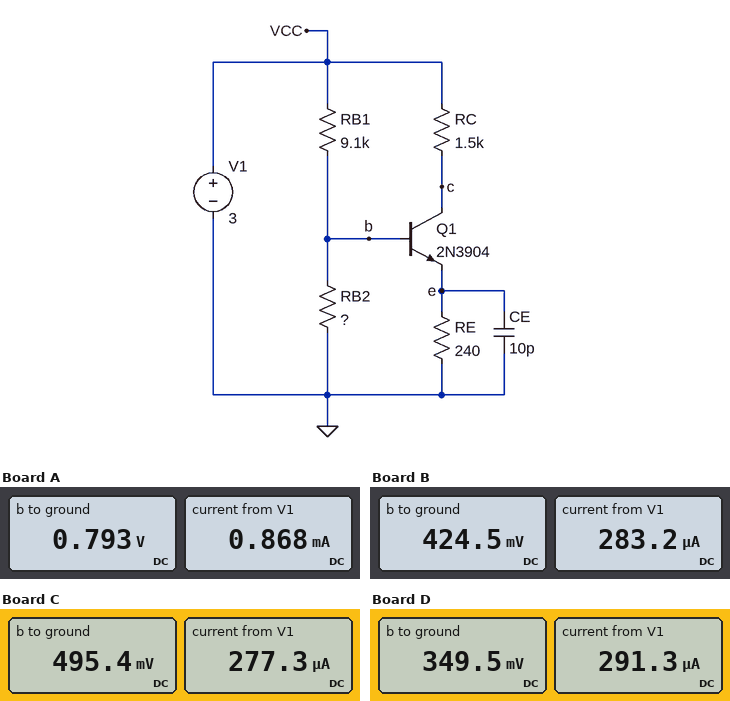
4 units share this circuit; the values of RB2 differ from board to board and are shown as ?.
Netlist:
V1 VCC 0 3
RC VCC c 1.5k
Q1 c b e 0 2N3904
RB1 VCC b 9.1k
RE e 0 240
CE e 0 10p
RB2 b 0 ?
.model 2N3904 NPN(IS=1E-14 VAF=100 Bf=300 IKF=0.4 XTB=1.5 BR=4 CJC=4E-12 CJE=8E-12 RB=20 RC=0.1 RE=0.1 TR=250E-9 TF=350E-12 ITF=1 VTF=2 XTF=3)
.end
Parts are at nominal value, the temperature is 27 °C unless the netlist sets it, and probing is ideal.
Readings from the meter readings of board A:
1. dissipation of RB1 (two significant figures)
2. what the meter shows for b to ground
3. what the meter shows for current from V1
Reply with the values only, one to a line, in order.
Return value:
540 µW
0.793 V
0.868 mA
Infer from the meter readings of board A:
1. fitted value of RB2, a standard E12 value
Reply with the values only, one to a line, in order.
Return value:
3.3 kΩ
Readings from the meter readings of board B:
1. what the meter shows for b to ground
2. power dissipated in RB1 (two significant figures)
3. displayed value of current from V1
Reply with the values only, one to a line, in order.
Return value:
424.5 mV
730 µW
283.2 µA
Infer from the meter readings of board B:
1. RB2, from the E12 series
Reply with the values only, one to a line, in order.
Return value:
1.5 kΩ
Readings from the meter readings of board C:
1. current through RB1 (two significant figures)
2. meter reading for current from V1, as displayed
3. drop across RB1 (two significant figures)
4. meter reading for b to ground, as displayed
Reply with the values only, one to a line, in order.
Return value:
280 µA
277.3 µA
2.5 V
495.4 mV
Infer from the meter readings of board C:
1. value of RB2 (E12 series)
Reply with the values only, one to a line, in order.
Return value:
1.8 kΩ
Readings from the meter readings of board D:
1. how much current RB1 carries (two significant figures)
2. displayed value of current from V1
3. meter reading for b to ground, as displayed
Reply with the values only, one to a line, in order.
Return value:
290 µA
291.3 µA
349.5 mV
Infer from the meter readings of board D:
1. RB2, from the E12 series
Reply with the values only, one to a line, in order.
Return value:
1.2 kΩ
